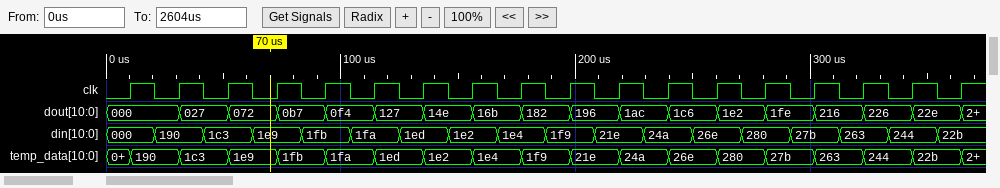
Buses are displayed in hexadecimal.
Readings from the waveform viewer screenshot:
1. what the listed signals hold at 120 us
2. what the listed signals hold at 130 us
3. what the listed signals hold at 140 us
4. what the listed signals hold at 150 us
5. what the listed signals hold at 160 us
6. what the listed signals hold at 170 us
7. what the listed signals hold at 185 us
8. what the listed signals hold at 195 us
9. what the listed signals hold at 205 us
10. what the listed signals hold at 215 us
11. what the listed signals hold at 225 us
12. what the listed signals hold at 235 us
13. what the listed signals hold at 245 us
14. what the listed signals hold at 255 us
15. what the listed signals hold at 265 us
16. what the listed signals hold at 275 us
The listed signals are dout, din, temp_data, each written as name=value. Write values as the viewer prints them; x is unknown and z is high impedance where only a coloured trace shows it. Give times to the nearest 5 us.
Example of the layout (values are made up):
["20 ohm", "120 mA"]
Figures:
["dout=127, din=1fa, temp_data=1ed", "dout=127, din=1ed, temp_data=1ed", "dout=14e, din=1ed, temp_data=1e2", "dout=14e, din=1e2, temp_data=1e2", "dout=16b, din=1e2, temp_data=1e4", "dout=16b, din=1e4, temp_data=1e4", "dout=182, din=1e4, temp_data=1f9", "dout=182, din=1f9, temp_data=1f9", "dout=196, din=1f9, temp_data=21e", "dout=196, din=21e, temp_data=21e", "dout=1ac, din=21e, temp_data=24a", "dout=1ac, din=24a, temp_data=24a", "dout=1c6, din=24a, temp_data=26e", "dout=1c6, din=26e, temp_data=26e", "dout=1e2, din=26e, temp_data=280", "dout=1e2, din=280, temp_data=280"]
